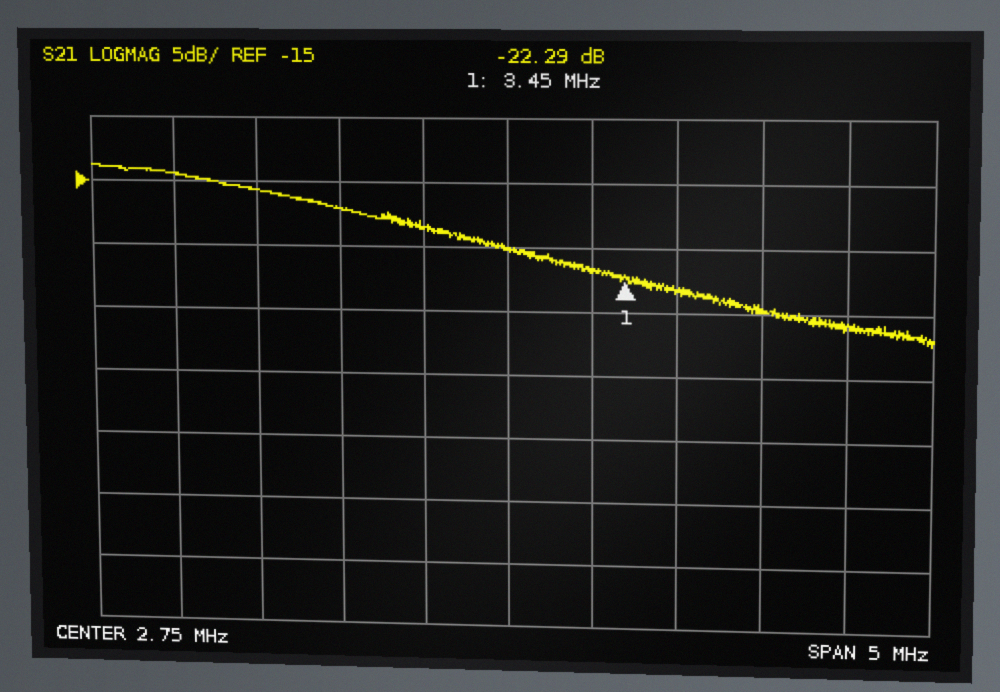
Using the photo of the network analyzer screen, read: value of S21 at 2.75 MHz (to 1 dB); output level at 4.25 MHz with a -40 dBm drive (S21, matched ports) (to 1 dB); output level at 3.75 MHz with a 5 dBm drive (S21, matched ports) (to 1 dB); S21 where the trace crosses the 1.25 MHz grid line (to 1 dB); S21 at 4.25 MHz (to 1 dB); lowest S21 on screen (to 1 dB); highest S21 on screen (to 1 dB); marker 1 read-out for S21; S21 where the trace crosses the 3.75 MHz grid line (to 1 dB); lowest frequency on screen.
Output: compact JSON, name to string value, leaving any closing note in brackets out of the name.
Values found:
{"value of S21 at 2.75 MHz": "-20 dB", "output level at 4.25 MHz with a -40 dBm drive (S21, matched ports)": "-65 dBm", "output level at 3.75 MHz with a 5 dBm drive (S21, matched ports)": "-18 dBm", "S21 where the trace crosses the 1.25 MHz grid line": "-16 dB", "S21 at 4.25 MHz": "-25 dB", "lowest S21 on screen": "-27 dB", "highest S21 on screen": "-14 dB", "marker 1 read-out for S21": "-22.29 dB", "S21 where the trace crosses the 3.75 MHz grid line": "-23 dB", "lowest frequency on screen": "250 kHz"}
